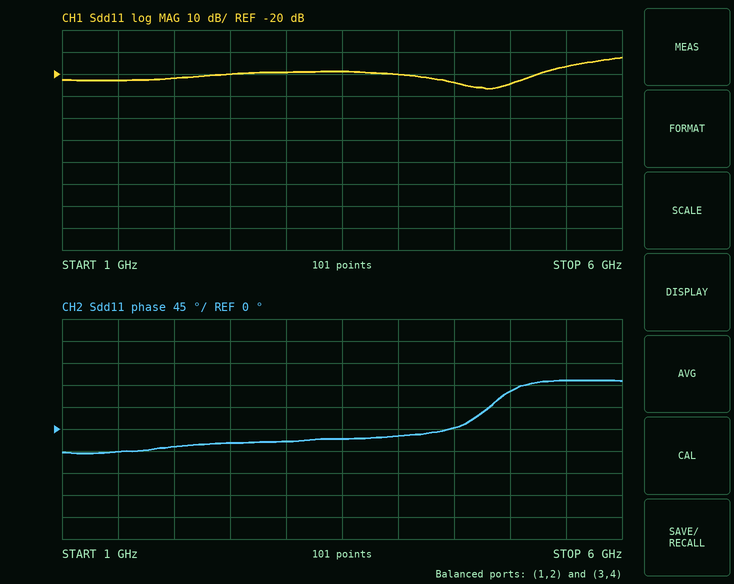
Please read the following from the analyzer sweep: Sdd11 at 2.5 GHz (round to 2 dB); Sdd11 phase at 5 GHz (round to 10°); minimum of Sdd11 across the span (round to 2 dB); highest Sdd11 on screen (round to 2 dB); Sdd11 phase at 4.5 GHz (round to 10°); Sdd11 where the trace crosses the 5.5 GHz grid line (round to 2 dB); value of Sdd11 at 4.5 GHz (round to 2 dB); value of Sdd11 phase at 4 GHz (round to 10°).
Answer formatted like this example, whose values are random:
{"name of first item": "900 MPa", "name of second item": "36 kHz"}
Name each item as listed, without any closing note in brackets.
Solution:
{"Sdd11 at 2.5 GHz": "-20 dB", "Sdd11 phase at 5 GHz": "80°", "minimum of Sdd11 across the span": "-26 dB", "highest Sdd11 on screen": "-12 dB", "Sdd11 phase at 4.5 GHz": "0°", "Sdd11 where the trace crosses the 5.5 GHz grid line": "-16 dB", "value of Sdd11 at 4.5 GHz": "-24 dB", "value of Sdd11 phase at 4 GHz": "-10°"}
